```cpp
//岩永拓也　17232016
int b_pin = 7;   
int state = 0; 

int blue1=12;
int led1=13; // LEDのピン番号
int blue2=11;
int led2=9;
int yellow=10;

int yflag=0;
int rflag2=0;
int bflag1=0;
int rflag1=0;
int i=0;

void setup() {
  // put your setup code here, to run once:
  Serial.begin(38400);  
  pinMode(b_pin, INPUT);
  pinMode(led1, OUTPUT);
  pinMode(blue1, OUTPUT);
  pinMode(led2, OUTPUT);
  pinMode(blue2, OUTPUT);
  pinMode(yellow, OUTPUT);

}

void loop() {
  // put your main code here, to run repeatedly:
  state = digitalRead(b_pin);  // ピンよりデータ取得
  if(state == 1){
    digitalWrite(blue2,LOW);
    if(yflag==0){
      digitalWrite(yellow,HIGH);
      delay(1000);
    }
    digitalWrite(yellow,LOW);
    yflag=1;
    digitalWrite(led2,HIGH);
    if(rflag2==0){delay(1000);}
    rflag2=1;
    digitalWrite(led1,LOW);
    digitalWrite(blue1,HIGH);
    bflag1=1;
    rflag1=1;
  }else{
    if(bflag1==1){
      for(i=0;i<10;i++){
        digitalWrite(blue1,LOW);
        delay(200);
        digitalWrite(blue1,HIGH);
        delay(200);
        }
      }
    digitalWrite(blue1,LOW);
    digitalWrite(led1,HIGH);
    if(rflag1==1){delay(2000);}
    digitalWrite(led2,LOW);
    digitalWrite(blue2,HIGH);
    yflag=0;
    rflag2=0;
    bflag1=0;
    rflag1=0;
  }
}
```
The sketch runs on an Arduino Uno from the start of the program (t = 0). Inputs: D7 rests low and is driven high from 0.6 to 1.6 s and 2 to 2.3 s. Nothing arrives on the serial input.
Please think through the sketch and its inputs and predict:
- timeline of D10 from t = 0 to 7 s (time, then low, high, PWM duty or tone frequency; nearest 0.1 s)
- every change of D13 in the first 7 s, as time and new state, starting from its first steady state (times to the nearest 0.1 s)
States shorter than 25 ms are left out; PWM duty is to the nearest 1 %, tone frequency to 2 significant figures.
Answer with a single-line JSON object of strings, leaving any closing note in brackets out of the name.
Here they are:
{"timeline of D10 from t = 0 to 7 s": "0 s low; 0.6 s high; 1.6 s low", "every change of D13 in the first 7 s, as time and new state, starting from its first steady state": "0 s high; 2.6 s low; 6.6 s high"}
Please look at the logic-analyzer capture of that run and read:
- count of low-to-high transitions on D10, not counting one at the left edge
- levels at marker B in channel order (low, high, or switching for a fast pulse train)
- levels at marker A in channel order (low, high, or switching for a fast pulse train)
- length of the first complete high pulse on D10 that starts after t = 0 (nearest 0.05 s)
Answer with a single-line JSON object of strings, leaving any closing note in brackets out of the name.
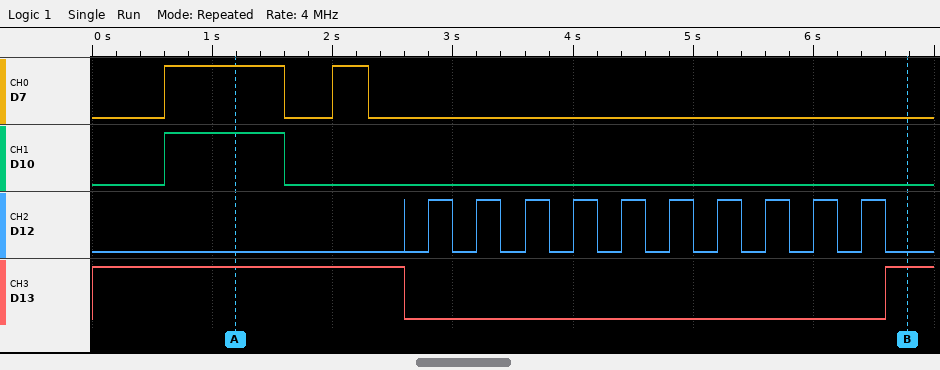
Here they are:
{"count of low-to-high transitions on D10, not counting one at the left edge": "1", "levels at marker B in channel order": "D7 low, D10 low, D12 low, D13 high", "levels at marker A in channel order": "D7 high, D10 high, D12 low, D13 high", "length of the first complete high pulse on D10 that starts after t = 0": "1.00 s"}
